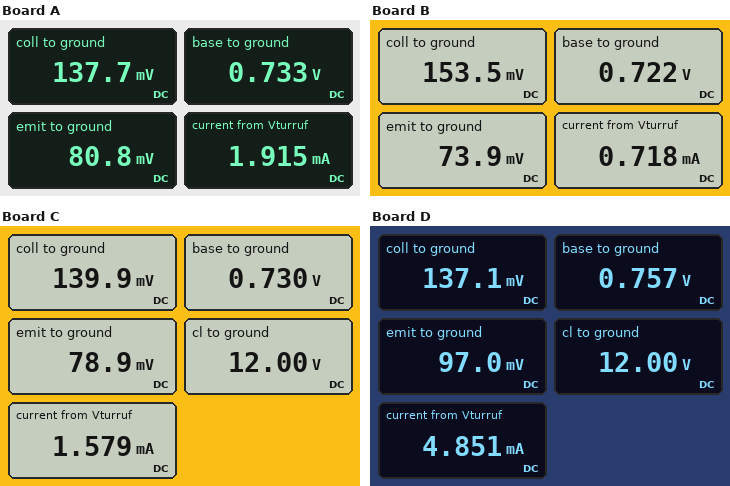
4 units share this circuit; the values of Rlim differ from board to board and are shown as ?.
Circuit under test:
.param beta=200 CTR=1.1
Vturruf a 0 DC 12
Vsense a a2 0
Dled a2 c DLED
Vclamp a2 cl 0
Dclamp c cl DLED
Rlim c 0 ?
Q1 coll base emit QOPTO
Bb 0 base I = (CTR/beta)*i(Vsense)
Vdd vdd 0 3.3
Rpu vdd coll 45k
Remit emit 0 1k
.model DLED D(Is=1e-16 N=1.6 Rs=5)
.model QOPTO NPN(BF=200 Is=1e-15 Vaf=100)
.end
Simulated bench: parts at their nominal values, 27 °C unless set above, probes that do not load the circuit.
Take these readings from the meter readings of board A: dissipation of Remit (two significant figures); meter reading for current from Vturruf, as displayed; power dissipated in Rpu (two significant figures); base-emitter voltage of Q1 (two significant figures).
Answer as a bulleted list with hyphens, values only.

- 6.5 µW
- 1.915 mA
- 220 µW
- 650 mV
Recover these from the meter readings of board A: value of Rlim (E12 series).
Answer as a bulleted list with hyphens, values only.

- 5.6 kΩ
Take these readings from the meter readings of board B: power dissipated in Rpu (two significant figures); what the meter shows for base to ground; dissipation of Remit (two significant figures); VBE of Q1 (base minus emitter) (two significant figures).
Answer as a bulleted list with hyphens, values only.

- 220 µW
- 0.722 V
- 5.5 µW
- 650 mV
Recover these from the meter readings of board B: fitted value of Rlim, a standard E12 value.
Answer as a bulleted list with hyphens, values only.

- 15 kΩ
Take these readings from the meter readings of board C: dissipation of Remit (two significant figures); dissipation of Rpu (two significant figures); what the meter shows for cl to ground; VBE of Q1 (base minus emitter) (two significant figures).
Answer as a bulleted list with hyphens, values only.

- 6.2 µW
- 220 µW
- 12.00 V
- 650 mV
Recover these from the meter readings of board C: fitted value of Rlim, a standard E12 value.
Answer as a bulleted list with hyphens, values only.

- 6.8 kΩ
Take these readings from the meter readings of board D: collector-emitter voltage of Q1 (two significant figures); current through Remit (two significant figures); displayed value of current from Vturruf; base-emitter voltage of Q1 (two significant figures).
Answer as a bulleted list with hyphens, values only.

- 40 mV
- 97 µA
- 4.851 mA
- 660 mV
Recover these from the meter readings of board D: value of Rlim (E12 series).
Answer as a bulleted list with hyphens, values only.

- 2.2 kΩ
